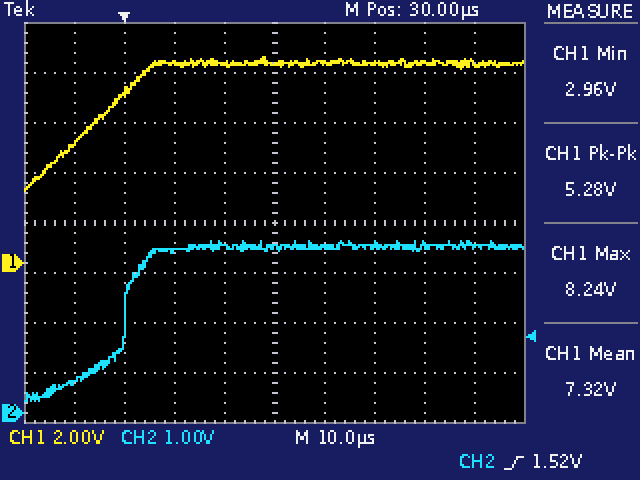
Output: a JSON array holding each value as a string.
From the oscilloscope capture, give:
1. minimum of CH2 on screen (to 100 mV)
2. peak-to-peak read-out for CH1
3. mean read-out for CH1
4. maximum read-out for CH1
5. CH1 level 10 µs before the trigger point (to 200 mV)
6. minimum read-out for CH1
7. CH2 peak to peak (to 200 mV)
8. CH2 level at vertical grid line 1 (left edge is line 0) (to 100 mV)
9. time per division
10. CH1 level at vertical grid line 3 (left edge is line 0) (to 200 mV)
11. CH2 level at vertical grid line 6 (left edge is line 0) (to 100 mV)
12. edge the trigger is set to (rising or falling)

["200 mV", "5.28 V", "7.32 V", "8.24 V", "4.8 V", "2.96 V", "3.2 V", "600 mV", "10 µs", "8.0 V", "3.3 V", "rising"]
